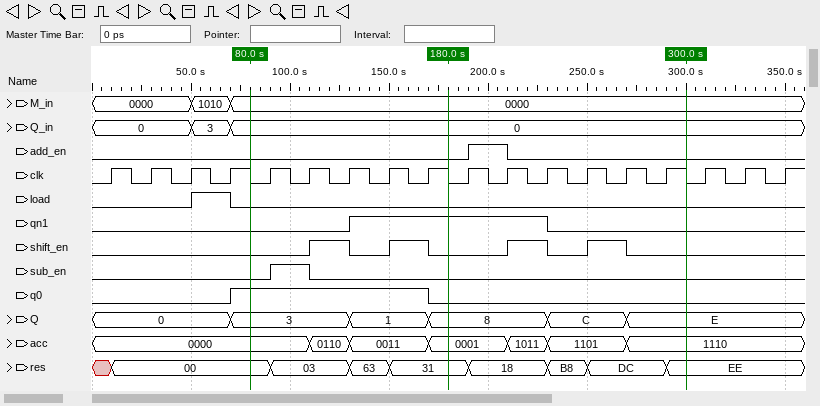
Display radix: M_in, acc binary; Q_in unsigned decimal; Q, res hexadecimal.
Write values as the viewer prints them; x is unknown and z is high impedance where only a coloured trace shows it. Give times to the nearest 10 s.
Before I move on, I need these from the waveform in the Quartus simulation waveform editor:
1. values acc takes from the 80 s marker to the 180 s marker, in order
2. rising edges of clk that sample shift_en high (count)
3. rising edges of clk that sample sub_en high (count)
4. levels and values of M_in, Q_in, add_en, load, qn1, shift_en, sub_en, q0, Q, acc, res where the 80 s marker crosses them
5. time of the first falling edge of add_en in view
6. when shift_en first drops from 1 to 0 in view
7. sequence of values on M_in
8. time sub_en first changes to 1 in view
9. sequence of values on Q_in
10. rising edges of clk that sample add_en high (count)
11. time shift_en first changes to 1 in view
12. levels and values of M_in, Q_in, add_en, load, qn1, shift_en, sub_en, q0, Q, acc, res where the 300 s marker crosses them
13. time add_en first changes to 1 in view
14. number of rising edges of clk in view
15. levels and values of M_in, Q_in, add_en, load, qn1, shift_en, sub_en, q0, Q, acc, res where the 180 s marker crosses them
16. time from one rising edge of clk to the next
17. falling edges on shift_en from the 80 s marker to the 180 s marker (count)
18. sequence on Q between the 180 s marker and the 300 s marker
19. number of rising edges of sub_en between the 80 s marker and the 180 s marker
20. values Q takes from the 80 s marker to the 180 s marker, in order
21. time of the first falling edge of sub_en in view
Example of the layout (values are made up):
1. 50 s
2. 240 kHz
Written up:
1. 0000, 0110, 0011, 0001
2. 4
3. 1
4. M_in=0000, Q_in=0, add_en=0, load=0, qn1=0, shift_en=0, sub_en=0, q0=1, Q=3, acc=0000, res=00
5. 210 s
6. 130 s
7. 0000, 1010, 0000
8. 90 s
9. 0, 3, 0
10. 1
11. 110 s
12. M_in=0000, Q_in=0, add_en=0, load=0, qn1=0, shift_en=0, sub_en=0, q0=0, Q=E, acc=1110, res=EE
13. 190 s
14. 18
15. M_in=0000, Q_in=0, add_en=0, load=0, qn1=1, shift_en=0, sub_en=0, q0=0, Q=8, acc=0001, res=31
16. 20 s
17. 2
18. 8, C, E
19. 1
20. 3, 1, 8
21. 110 s
